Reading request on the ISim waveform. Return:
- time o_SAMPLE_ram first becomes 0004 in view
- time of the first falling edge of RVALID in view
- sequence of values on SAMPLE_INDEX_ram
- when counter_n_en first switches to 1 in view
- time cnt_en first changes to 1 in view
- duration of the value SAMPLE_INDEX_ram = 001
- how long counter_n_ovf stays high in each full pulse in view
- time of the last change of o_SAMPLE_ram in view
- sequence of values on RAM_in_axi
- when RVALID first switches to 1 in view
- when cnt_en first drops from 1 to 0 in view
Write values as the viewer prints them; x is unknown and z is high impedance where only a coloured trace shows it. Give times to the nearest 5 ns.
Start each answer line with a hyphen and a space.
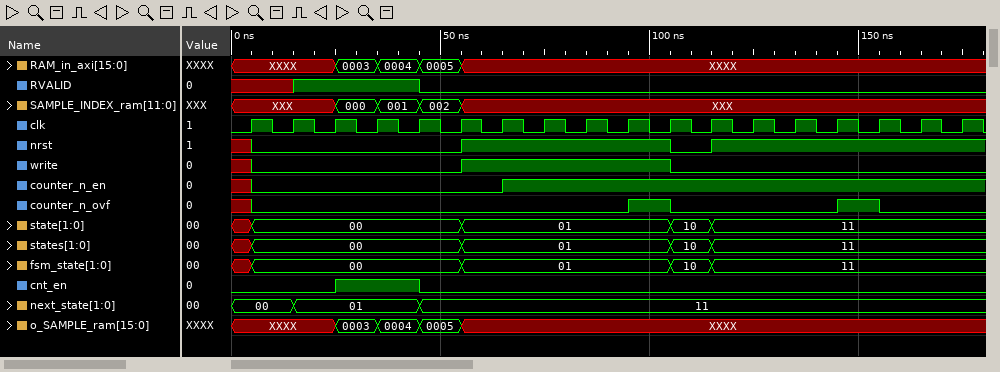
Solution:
- 35 ns
- 45 ns
- XXX, 000, 001, 002, XXX
- 65 ns
- 25 ns
- 10 ns
- 10 ns, 10 ns
- 55 ns
- XXXX, 0003, 0004, 0005, XXXX
- 15 ns
- 45 ns
